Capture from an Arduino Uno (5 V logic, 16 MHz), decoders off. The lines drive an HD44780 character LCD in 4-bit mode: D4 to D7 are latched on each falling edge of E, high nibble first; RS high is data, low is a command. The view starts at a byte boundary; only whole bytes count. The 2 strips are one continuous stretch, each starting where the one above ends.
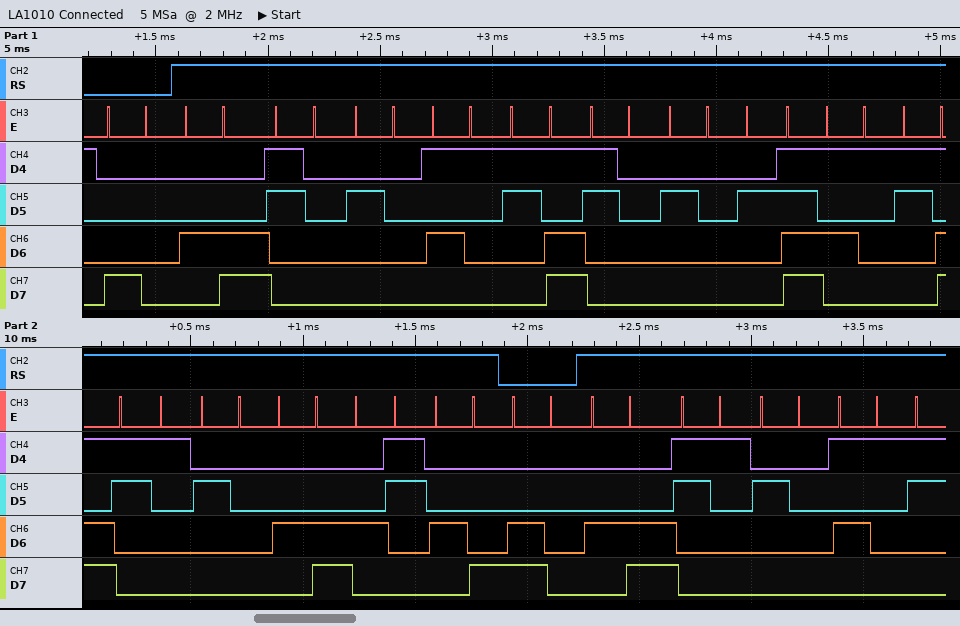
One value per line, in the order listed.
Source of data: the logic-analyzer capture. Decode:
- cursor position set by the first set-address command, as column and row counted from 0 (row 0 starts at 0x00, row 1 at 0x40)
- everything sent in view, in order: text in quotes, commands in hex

column 0, row 0
0x80 "L0 Q=0 /Q=1 LCH" 0xC0 "L1 Q"
